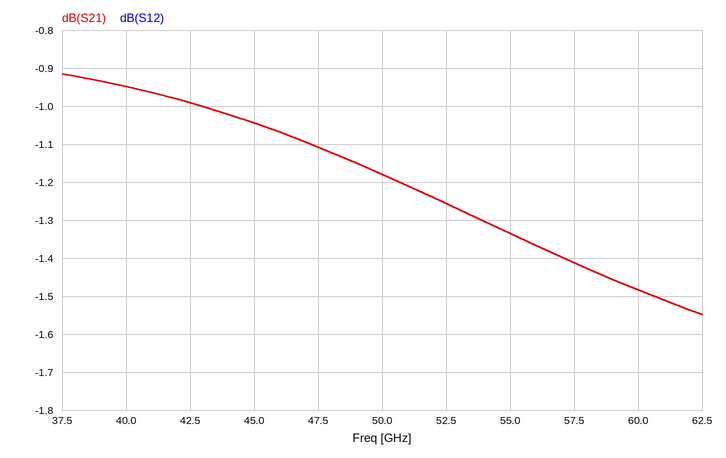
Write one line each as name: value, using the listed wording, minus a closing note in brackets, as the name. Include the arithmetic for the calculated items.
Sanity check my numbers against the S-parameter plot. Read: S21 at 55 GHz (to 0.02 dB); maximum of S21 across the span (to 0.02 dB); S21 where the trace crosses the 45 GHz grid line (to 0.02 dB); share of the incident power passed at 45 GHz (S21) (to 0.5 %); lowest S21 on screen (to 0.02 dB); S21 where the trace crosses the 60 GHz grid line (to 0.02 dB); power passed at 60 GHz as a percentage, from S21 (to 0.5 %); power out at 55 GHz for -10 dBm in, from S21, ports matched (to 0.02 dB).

S21 at 55 GHz: -1.34 dB
maximum of S21 across the span: -0.92 dB
S21 where the trace crosses the 45 GHz grid line: -1.04 dB
share of the incident power passed at 45 GHz (S21): 10^(-1.04/10) ≈ 78.7 %, so 78.5 % to the nearest 0.5 %
lowest S21 on screen: -1.54 dB
S21 where the trace crosses the 60 GHz grid line: -1.48 dB
power passed at 60 GHz as a percentage, from S21: 10^(-1.48/10) ≈ 71.1 %, so 71.0 % to the nearest 0.5 %
power out at 55 GHz for -10 dBm in, from S21, ports matched: -10 dBm + (-1.34 dB) = -11.34 dBm
